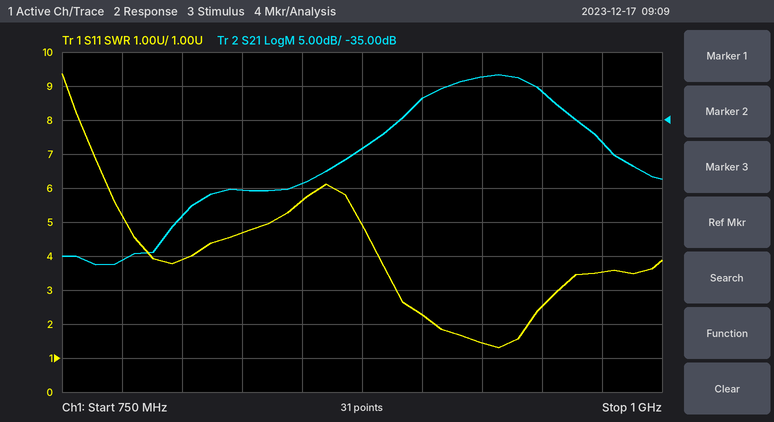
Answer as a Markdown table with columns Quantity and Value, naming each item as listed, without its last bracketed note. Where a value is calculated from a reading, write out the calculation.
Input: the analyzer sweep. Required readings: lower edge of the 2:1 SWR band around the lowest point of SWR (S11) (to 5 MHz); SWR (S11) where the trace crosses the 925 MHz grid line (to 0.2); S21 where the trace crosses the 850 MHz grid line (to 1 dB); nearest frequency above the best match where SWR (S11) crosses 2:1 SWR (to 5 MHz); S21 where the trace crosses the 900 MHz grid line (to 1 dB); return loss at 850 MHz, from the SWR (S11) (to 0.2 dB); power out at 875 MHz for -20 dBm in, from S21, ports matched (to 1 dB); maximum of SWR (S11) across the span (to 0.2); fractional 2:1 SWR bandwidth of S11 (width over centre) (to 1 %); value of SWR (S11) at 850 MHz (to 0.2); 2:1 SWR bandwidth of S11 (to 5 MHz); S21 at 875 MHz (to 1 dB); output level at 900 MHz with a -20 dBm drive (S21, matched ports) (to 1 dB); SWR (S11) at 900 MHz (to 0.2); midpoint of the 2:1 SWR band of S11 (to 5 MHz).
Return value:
| Quantity | Value |
|---|---|
| lower edge of the 2:1 SWR band around the lowest point of SWR (S11) | 905 MHz |
| SWR (S11) where the trace crosses the 925 MHz grid line | 1.4 |
| S21 where the trace crosses the 850 MHz grid line | -44 dB |
| nearest frequency above the best match where SWR (S11) crosses 2:1 SWR | 945 MHz |
| S21 where the trace crosses the 900 MHz grid line | -32 dB |
| return loss at 850 MHz, from the SWR (S11) | −20 log10((5.6 − 1)/(5.6 + 1)) ≈ 3.14 dB, so 3.2 dB to the nearest 0.2 dB |
| power out at 875 MHz for -20 dBm in, from S21, ports matched | -20 dBm + (-39 dB) = -59 dBm |
| maximum of SWR (S11) across the span | 9.4 |
| fractional 2:1 SWR bandwidth of S11 (width over centre) | 40 MHz / 925 MHz ≈ 4 % |
| value of SWR (S11) at 850 MHz | 5.6 |
| 2:1 SWR bandwidth of S11 | 945 MHz − 905 MHz = 40 MHz |
| S21 at 875 MHz | -39 dB |
| output level at 900 MHz with a -20 dBm drive (S21, matched ports) | -20 dBm + (-32 dB) = -52 dBm |
| SWR (S11) at 900 MHz | 2.2 |
| midpoint of the 2:1 SWR band of S11 | 925 MHz |
